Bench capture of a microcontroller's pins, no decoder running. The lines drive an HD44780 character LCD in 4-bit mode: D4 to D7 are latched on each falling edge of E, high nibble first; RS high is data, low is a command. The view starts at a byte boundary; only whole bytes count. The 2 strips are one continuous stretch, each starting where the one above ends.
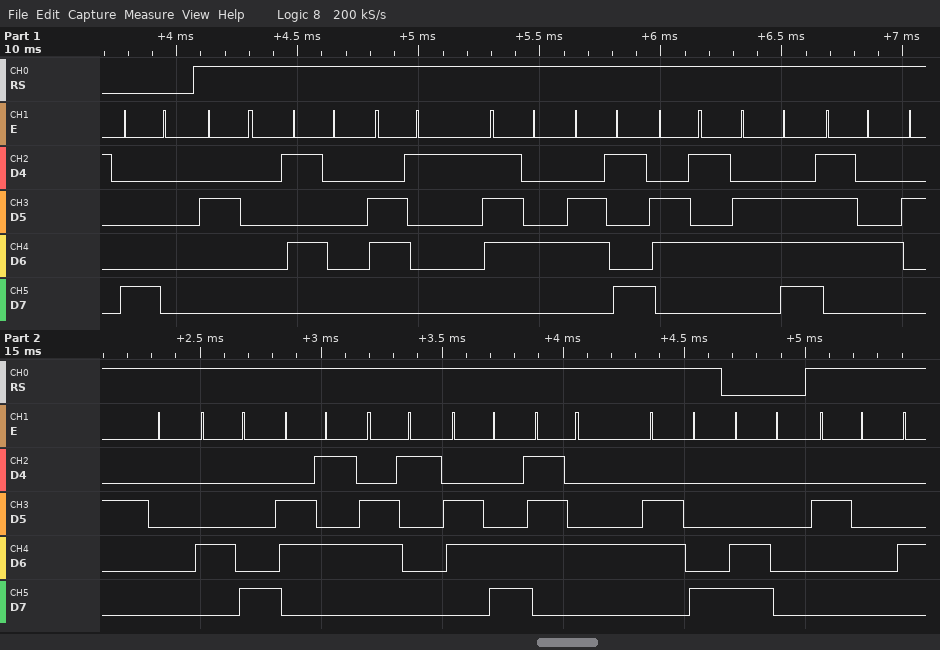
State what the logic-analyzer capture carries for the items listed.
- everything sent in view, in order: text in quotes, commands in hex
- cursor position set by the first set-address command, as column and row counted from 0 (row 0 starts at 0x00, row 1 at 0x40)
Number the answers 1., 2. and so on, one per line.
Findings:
1. 0x80 " Patient Health" 0xC0 " "
2. column 0, row 0
